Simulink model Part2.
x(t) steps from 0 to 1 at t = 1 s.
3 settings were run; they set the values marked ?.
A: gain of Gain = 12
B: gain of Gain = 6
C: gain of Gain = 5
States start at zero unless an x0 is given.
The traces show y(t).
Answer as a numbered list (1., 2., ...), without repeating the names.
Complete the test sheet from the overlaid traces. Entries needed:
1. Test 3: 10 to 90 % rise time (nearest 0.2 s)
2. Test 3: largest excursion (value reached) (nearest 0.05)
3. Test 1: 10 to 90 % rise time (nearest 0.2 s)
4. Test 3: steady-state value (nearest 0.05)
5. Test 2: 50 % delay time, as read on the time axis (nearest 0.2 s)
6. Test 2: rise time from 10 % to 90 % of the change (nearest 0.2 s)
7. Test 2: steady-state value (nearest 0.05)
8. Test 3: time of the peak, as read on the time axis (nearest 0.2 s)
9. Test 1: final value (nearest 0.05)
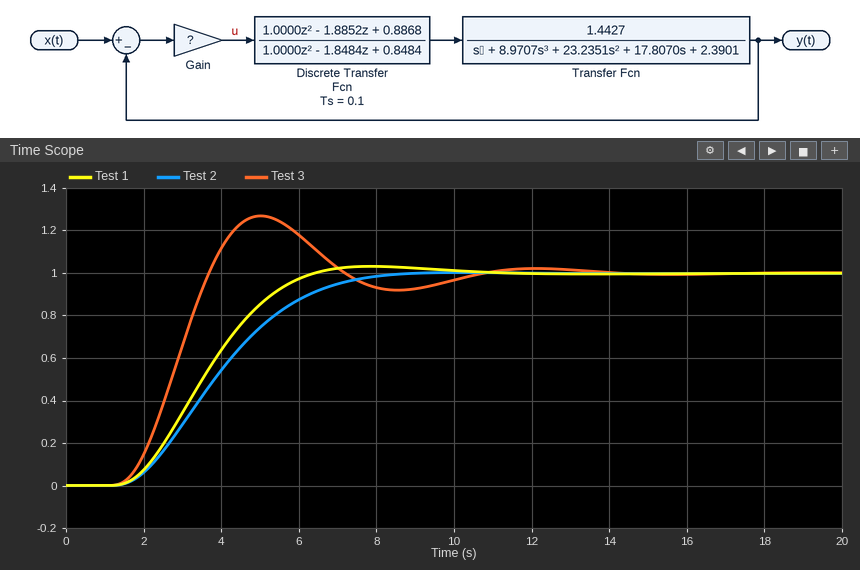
1. 1.6 s
2. 1.25
3. 3.2 s
4. 1.00
5. 3.8 s
6. 4.0 s
7. 1.00
8. 5.0 s
9. 1.00
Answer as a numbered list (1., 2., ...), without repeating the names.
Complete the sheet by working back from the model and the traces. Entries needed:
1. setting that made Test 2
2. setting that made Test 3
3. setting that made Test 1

1. C
2. A
3. B
